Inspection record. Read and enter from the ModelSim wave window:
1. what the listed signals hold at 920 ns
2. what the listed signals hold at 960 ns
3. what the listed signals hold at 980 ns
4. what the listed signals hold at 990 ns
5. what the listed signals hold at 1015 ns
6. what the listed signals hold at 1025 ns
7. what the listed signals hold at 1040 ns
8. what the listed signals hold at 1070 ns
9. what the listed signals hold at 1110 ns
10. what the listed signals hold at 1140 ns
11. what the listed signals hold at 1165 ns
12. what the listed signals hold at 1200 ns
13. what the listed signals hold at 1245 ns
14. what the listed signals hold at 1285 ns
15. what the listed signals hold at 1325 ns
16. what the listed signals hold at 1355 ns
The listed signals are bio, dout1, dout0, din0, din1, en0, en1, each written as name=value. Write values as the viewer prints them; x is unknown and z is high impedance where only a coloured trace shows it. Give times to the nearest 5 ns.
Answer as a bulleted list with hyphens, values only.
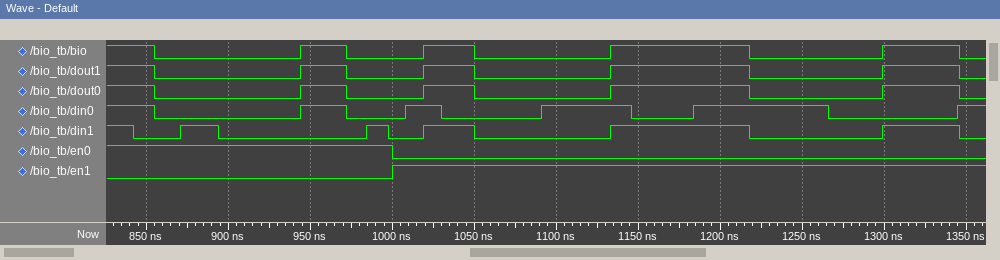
- bio=0, dout1=0, dout0=0, din0=0, din1=0, en0=1, en1=0
- bio=1, dout1=1, dout0=1, din0=1, din1=0, en0=1, en1=0
- bio=0, dout1=0, dout0=0, din0=0, din1=0, en0=1, en1=0
- bio=0, dout1=0, dout0=0, din0=0, din1=1, en0=1, en1=0
- bio=0, dout1=0, dout0=0, din0=1, din1=0, en0=0, en1=1
- bio=1, dout1=1, dout0=1, din0=1, din1=1, en0=0, en1=1
- bio=1, dout1=1, dout0=1, din0=0, din1=1, en0=0, en1=1
- bio=0, dout1=0, dout0=0, din0=0, din1=0, en0=0, en1=1
- bio=0, dout1=0, dout0=0, din0=1, din1=0, en0=0, en1=1
- bio=1, dout1=1, dout0=1, din0=1, din1=1, en0=0, en1=1
- bio=1, dout1=1, dout0=1, din0=0, din1=1, en0=0, en1=1
- bio=1, dout1=1, dout0=1, din0=1, din1=1, en0=0, en1=1
- bio=0, dout1=0, dout0=0, din0=1, din1=0, en0=0, en1=1
- bio=0, dout1=0, dout0=0, din0=0, din1=0, en0=0, en1=1
- bio=1, dout1=1, dout0=1, din0=0, din1=1, en0=0, en1=1
- bio=0, dout1=0, dout0=0, din0=1, din1=0, en0=0, en1=1
